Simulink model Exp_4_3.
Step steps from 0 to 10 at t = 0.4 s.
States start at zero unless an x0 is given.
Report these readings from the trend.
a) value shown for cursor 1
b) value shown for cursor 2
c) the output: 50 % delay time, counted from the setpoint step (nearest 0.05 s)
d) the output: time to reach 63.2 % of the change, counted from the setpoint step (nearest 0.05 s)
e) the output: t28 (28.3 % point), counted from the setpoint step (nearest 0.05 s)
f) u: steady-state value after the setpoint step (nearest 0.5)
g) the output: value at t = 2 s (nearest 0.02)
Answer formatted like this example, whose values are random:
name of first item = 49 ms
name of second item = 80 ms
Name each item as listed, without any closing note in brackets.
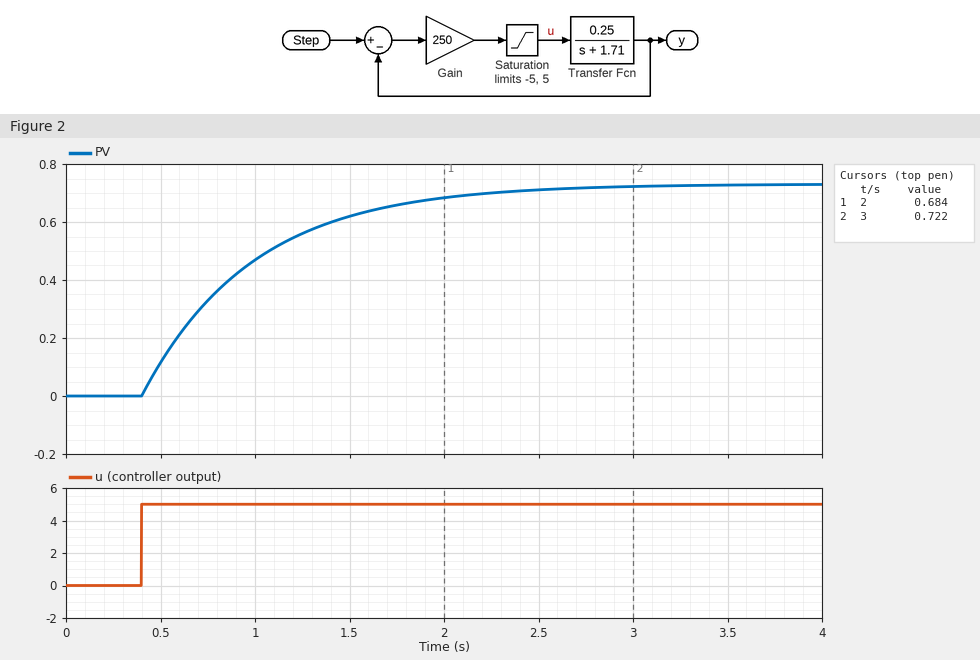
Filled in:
value shown for cursor 1 = 0.684
value shown for cursor 2 = 0.722
the output: 50 % delay time, counted from the setpoint step = 0.40 s
the output: time to reach 63.2 % of the change, counted from the setpoint step = 0.60 s
the output: t28 (28.3 % point), counted from the setpoint step = 0.20 s
u: steady-state value after the setpoint step = 5.0
the output: value at t = 2 s = 0.68
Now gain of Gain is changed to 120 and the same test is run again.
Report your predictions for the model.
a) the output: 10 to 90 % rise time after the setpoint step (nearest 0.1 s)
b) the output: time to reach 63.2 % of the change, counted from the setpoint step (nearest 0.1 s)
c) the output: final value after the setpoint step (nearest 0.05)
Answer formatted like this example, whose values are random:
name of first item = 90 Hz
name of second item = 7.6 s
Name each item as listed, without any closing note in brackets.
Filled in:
the output: 10 to 90 % rise time after the setpoint step = 1.3 s
the output: time to reach 63.2 % of the change, counted from the setpoint step = 0.6 s
the output: final value after the setpoint step = 0.75
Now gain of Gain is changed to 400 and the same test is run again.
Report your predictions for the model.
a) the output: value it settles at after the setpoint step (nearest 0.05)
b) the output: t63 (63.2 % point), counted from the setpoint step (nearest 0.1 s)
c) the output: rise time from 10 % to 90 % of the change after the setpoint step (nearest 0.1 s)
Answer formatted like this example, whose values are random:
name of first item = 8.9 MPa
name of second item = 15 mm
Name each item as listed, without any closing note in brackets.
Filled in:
the output: value it settles at after the setpoint step = 0.75
the output: t63 (63.2 % point), counted from the setpoint step = 0.6 s
the output: rise time from 10 % to 90 % of the change after the setpoint step = 1.3 s
